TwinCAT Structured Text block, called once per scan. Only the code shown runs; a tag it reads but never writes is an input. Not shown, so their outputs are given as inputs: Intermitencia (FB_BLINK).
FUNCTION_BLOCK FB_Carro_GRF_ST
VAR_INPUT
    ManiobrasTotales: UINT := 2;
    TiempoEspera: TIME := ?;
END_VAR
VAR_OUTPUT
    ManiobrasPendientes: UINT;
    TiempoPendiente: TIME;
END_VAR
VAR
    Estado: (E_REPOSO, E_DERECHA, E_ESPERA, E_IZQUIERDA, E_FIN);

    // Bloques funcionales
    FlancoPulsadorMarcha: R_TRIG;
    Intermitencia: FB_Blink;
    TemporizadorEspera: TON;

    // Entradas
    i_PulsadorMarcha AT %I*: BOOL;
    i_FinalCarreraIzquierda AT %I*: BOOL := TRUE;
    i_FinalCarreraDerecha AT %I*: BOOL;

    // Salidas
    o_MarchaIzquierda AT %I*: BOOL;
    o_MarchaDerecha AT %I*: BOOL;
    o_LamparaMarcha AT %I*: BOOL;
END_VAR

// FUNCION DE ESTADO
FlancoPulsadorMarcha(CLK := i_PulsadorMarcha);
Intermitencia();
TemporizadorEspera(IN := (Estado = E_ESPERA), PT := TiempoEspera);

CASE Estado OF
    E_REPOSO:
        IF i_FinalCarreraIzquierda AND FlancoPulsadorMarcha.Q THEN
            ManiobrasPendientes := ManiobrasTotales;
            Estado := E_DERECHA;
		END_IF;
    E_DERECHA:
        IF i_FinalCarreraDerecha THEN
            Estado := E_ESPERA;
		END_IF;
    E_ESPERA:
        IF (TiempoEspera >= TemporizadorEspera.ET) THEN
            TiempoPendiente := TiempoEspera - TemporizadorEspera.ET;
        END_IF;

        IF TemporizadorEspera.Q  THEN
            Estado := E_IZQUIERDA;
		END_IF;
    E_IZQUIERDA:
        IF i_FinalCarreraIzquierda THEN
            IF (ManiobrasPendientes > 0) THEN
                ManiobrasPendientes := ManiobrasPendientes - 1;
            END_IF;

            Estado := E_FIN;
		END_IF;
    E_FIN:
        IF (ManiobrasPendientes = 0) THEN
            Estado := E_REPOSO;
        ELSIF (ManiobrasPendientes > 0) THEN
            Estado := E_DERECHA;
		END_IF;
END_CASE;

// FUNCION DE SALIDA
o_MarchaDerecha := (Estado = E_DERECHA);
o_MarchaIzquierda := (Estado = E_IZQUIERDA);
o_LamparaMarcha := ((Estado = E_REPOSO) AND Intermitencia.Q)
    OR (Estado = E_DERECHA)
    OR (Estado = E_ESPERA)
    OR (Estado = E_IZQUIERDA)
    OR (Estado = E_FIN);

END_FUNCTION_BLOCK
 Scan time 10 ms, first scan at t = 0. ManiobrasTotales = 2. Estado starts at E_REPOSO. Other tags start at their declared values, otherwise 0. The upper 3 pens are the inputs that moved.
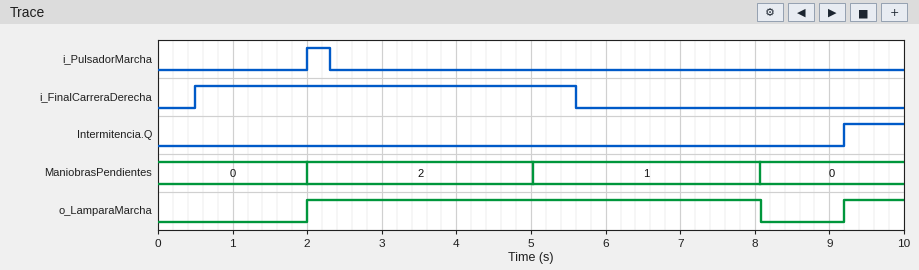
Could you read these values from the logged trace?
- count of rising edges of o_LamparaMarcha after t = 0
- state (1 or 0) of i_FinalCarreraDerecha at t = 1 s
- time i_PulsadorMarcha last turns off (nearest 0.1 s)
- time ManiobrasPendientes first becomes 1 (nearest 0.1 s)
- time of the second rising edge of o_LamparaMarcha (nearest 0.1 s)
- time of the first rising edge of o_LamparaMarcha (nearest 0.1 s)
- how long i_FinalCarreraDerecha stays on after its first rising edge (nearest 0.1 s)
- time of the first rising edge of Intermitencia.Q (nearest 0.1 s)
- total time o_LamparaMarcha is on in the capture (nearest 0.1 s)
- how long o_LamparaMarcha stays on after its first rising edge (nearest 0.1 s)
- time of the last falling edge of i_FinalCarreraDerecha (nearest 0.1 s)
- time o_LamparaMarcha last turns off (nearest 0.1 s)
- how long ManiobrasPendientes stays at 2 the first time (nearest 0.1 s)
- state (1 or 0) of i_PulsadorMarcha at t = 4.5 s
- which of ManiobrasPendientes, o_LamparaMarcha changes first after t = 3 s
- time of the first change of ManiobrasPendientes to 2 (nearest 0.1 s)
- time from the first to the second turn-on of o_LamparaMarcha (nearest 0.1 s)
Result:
2
1
2.3 s
5.0 s
9.2 s
2.0 s
5.1 s
9.2 s
6.9 s
6.1 s
5.6 s
8.1 s
3.0 s
0
ManiobrasPendientes
2.0 s
7.2 s
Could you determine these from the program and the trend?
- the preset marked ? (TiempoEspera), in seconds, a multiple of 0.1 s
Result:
3.0 s
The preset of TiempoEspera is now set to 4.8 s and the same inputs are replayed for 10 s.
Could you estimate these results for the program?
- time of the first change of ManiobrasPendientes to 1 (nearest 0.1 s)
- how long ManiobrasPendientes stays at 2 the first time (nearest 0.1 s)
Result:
6.8 s
4.8 s
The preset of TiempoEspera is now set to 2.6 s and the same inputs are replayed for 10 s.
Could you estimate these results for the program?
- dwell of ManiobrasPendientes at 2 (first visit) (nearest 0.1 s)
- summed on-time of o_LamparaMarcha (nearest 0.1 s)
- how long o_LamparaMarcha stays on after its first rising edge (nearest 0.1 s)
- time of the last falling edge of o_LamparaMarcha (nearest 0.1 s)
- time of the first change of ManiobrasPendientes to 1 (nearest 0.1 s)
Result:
2.6 s
6.1 s
5.3 s
7.3 s
4.6 s
